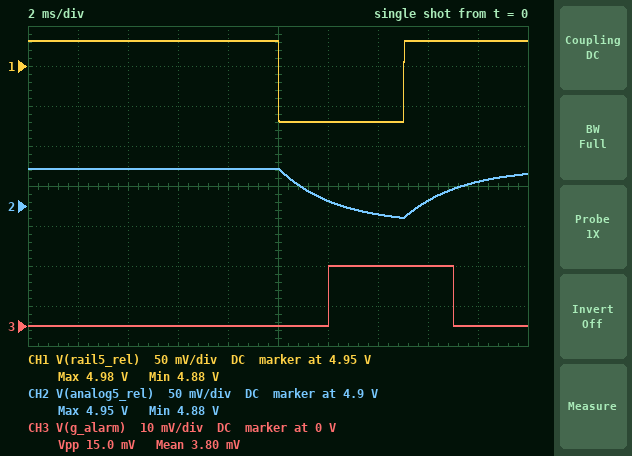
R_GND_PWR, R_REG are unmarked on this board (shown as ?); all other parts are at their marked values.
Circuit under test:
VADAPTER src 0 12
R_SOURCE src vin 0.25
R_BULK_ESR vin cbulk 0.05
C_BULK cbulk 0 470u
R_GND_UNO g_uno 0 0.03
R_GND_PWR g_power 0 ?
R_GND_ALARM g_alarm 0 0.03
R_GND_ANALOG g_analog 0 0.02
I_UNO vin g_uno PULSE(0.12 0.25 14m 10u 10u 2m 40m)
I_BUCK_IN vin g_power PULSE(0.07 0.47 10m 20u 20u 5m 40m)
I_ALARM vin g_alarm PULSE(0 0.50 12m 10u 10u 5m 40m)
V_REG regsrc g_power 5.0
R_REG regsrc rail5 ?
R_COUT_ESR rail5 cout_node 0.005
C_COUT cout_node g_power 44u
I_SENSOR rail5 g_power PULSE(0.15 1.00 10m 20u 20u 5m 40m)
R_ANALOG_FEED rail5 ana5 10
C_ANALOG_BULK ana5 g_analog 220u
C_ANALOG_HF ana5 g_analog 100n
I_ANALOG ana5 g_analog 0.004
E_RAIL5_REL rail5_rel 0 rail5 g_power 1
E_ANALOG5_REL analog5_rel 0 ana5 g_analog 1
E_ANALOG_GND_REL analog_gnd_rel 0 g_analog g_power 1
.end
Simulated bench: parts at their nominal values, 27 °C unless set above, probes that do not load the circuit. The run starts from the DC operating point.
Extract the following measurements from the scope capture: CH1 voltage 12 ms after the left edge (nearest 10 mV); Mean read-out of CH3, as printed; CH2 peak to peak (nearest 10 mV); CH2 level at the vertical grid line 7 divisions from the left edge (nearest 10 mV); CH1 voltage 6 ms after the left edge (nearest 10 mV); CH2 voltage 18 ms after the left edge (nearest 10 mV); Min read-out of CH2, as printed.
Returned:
4.88 V
3.80 mV
60 mV
4.89 V
4.98 V
4.93 V
4.88 V
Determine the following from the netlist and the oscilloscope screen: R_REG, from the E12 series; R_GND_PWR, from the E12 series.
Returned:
0.12 Ω
0.082 Ω
